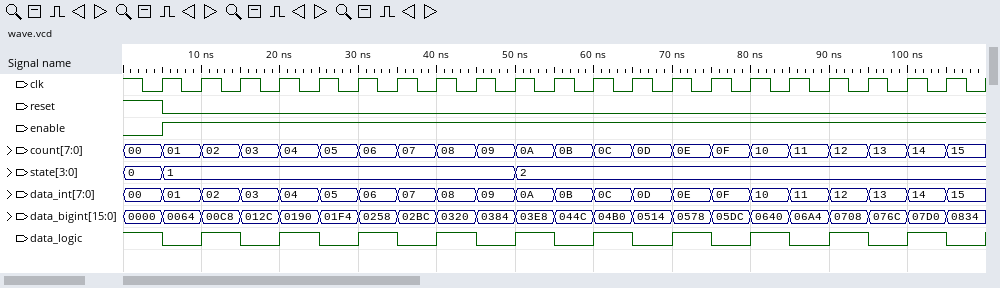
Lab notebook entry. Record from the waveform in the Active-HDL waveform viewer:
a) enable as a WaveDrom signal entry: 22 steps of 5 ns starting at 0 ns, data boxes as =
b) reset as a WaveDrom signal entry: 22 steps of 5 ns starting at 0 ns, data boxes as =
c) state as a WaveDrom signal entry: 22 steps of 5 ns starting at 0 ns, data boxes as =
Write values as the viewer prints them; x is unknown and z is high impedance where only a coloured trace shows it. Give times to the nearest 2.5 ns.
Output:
{name: 'enable', wave: '01....................'}
{name: 'reset', wave: '10....................'}
{name: 'state', wave: '==........=...........', data: '0 1 2'}
